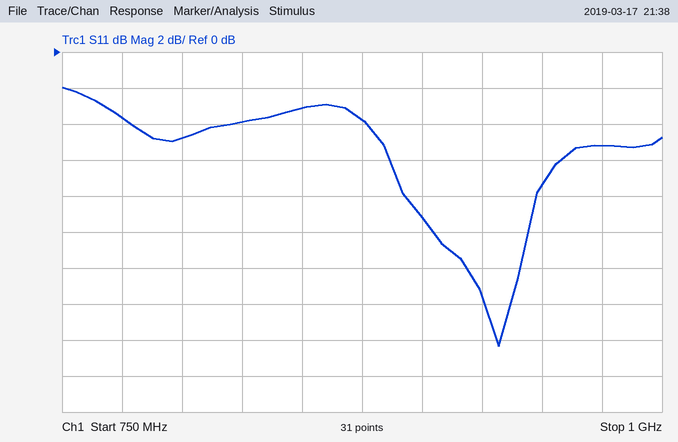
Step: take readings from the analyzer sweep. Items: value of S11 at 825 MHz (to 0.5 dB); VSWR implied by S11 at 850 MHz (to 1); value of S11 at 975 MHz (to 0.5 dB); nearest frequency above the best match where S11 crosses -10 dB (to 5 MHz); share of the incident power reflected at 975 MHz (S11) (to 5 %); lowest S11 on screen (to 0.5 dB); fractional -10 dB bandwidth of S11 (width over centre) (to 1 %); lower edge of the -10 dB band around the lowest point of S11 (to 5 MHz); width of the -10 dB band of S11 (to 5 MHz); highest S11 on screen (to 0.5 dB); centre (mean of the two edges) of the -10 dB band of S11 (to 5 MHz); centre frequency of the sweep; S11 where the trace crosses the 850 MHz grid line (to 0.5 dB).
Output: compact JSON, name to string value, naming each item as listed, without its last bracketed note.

{"value of S11 at 825 MHz": "-4.0 dB", "VSWR implied by S11 at 850 MHz": "6", "value of S11 at 975 MHz": "-5.0 dB", "nearest frequency above the best match where S11 crosses -10 dB": "945 MHz", "share of the incident power reflected at 975 MHz (S11)": "30 %", "lowest S11 on screen": "-16.5 dB", "fractional -10 dB bandwidth of S11 (width over centre)": "4 %", "lower edge of the -10 dB band around the lowest point of S11": "905 MHz", "width of the -10 dB band of S11": "40 MHz", "highest S11 on screen": "-2.0 dB", "centre (mean of the two edges) of the -10 dB band of S11": "925 MHz", "centre frequency of the sweep": "875 MHz", "S11 where the trace crosses the 850 MHz grid line": "-3.0 dB"}
